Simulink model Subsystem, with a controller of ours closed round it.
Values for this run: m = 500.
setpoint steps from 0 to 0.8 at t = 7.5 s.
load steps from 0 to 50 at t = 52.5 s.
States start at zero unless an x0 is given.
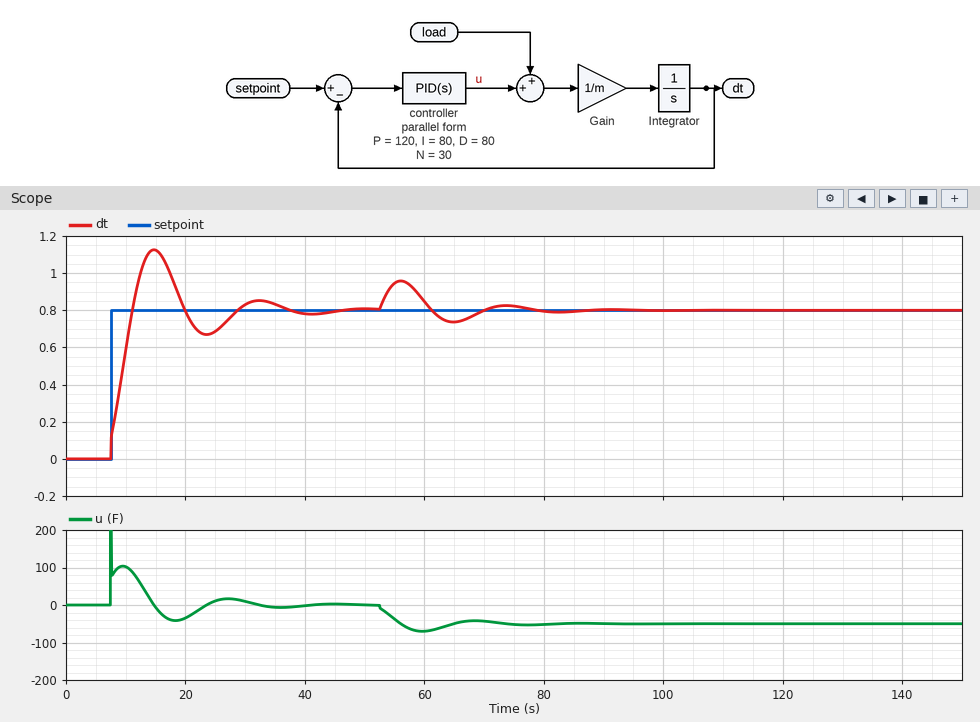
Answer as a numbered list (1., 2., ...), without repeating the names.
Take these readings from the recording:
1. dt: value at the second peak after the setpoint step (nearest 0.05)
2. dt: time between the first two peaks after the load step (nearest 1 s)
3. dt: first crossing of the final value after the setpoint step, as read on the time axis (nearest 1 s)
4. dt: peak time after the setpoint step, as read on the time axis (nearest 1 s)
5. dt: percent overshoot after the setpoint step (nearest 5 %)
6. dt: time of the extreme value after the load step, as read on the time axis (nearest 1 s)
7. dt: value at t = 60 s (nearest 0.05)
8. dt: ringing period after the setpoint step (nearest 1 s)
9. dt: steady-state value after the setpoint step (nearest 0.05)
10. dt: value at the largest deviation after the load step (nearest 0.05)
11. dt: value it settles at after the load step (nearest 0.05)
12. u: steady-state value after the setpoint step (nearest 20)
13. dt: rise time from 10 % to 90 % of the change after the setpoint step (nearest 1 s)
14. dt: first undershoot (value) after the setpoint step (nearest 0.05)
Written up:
1. 0.85
2. 18 s
3. 11 s
4. 15 s
5. 40 %
6. 56 s
7. 0.85
8. 18 s
9. 0.80
10. 0.95
11. 0.80
12. 0
13. 3 s
14. 0.65
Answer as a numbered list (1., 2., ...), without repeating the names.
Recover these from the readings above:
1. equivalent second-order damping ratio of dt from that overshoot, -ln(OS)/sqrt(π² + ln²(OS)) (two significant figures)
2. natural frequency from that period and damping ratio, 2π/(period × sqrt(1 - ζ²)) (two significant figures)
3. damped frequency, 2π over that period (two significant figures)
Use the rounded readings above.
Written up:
1. 0.28
2. 0.36 rad/s
3. 0.35 rad/s
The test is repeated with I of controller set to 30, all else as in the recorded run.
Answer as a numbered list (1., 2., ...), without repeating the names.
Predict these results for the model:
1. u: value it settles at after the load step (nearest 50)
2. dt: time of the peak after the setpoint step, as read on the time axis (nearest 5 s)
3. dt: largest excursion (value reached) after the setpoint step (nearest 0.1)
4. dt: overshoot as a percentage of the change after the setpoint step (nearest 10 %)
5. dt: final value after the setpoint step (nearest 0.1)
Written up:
1. -50
2. 20 s
3. 1.0
4. 30 %
5. 0.8
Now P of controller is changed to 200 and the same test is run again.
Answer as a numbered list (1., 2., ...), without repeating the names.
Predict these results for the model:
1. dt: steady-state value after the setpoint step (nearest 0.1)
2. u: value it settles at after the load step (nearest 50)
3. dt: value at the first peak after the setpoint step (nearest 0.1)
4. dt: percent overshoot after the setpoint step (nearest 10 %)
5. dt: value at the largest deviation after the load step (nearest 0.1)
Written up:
1. 0.8
2. -50
3. 1.0
4. 30 %
5. 0.9
